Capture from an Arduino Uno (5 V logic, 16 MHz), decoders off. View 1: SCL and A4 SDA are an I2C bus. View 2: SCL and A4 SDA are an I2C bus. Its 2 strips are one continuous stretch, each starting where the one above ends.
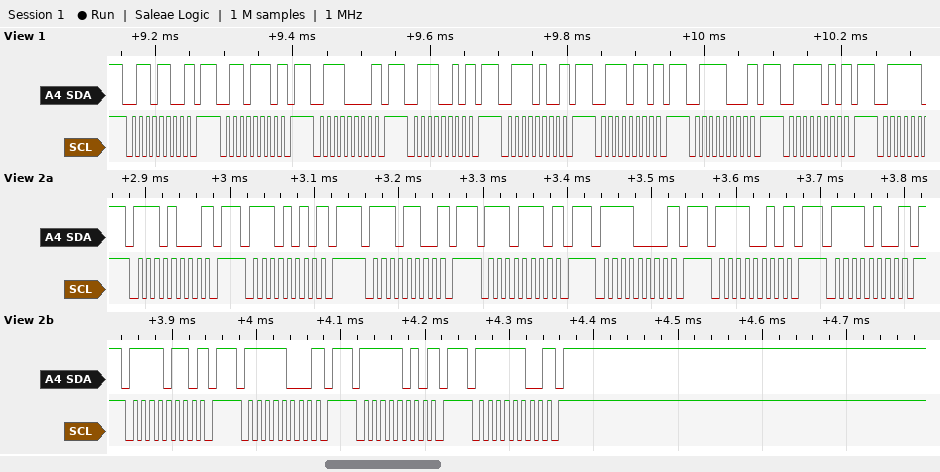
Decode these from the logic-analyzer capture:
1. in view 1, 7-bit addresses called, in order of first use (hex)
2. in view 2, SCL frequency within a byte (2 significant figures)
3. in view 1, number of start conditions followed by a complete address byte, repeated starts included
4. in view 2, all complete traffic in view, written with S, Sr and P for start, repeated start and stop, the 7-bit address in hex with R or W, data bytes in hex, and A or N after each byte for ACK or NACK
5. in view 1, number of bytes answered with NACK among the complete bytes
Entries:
0x36 0x37 0x38 0x39 0x3A 0x3B 0x3C 0x3D
100 kHz
8
S 74W N P S 75W N P S 76W N P S 77W N P S 78W N P S 79W N P S 7AW N P S 7BW N P S 7CW N P S 7DW N P S 7EW N P
8
